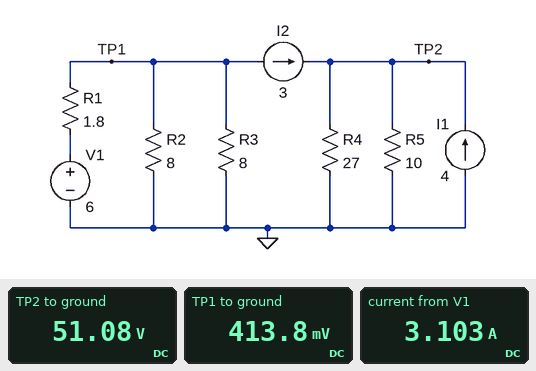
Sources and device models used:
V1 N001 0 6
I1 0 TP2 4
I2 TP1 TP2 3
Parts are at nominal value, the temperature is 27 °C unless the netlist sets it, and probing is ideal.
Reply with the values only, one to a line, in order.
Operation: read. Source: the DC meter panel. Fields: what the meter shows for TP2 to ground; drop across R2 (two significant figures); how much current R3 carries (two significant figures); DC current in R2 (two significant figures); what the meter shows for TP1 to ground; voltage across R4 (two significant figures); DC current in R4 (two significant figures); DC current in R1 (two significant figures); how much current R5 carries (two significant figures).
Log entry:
51.08 V
410 mV
52 mA
52 mA
413.8 mV
51 V
1.9 A
3.1 A
5.1 A
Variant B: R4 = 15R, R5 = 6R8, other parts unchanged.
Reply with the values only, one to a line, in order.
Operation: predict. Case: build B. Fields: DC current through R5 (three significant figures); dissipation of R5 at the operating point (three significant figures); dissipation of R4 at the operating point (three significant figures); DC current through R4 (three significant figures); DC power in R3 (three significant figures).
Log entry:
4.82 A
158 W
71.5 W
2.18 A
21.4 mW
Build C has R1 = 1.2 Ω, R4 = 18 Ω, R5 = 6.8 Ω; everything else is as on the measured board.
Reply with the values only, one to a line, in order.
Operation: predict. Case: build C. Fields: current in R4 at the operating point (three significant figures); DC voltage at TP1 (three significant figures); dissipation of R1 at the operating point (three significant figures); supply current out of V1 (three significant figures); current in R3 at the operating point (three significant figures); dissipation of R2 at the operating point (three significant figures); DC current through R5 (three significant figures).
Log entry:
1.92 A
1.85 V
14.4 W
3.46 A
231 mA
426 mW
5.08 A
